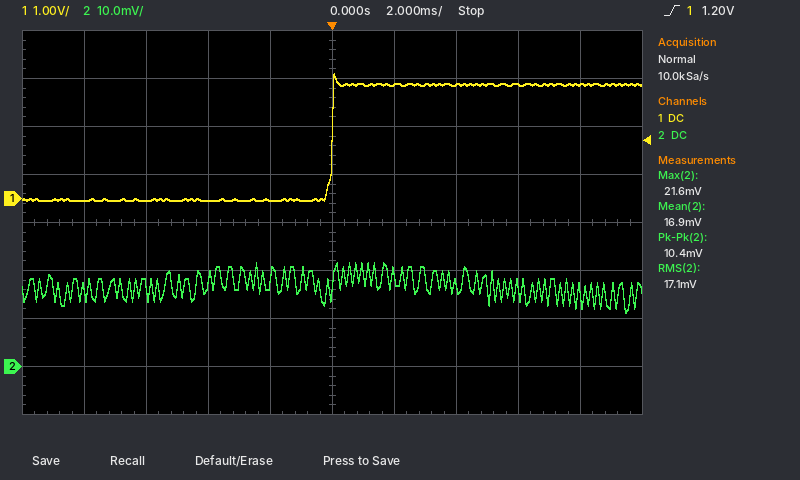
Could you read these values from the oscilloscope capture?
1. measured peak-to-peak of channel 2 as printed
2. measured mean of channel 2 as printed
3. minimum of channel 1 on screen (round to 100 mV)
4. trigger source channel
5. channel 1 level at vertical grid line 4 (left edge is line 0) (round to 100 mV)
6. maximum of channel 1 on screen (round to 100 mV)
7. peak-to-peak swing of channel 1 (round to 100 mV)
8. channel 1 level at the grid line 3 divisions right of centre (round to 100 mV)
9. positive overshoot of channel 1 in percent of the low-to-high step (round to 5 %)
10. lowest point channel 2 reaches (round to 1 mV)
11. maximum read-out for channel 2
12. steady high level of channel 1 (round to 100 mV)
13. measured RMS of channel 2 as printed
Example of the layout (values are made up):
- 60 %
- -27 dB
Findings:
- 10.4 mV
- 16.9 mV
- 0.0 V
- channel 1
- 0.0 V
- 2.6 V
- 2.6 V
- 2.4 V
- 10 %
- 11 mV
- 21.6 mV
- 2.4 V
- 17.1 mV
